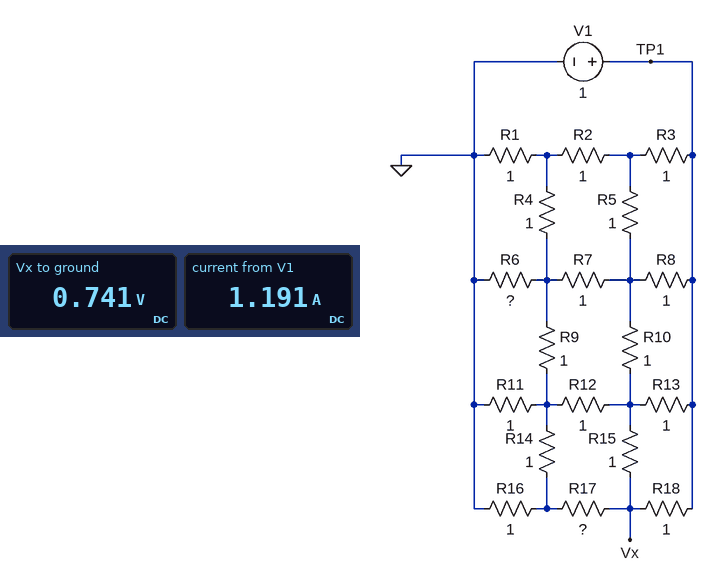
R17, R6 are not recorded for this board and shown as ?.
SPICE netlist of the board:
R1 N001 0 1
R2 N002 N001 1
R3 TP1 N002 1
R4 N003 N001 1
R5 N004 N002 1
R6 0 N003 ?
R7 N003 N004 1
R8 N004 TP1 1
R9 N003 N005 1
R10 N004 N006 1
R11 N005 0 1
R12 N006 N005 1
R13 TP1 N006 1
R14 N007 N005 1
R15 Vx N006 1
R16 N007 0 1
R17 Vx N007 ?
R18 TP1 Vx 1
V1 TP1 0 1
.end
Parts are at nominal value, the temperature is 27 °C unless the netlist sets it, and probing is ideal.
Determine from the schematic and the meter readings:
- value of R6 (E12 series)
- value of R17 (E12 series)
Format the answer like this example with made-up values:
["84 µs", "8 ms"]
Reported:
["1.8 Ω", "2.2 Ω"]
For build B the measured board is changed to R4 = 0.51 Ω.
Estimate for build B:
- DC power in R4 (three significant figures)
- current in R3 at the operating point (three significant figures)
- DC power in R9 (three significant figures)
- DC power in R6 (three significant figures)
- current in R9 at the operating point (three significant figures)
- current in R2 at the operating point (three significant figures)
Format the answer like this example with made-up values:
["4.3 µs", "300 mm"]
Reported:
["942 µW", "315 mA", "2.26 mW", "82.7 mW", "47.6 mA", "321 mA"]
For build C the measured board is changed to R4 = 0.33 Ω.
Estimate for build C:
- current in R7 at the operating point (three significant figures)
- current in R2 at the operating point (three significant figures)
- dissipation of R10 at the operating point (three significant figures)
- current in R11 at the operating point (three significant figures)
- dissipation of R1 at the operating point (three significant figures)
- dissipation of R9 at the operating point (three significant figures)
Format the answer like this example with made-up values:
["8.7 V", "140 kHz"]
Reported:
["307 mA", "319 mA", "2.98 µW", "337 mA", "135 mW", "2.09 mW"]
